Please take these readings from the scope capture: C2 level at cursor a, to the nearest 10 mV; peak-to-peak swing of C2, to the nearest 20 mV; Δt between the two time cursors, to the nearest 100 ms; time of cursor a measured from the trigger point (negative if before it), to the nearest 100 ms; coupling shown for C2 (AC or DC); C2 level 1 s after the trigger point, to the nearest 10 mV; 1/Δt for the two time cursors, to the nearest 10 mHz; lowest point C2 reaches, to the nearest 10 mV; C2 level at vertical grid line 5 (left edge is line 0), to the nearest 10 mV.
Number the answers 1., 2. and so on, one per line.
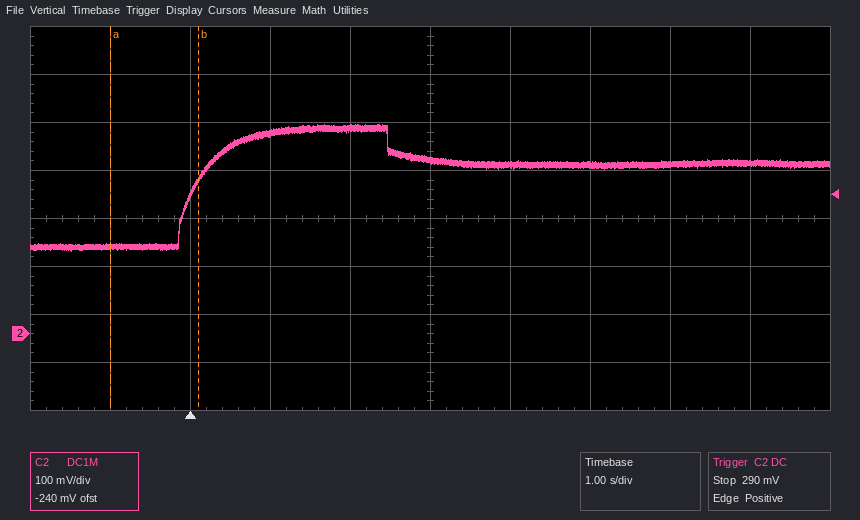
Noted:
1. 180 mV
2. 260 mV
3. 1.1 s
4. -1.0 s
5. DC
6. 420 mV
7. 910 mHz
8. 170 mV
9. 360 mV
